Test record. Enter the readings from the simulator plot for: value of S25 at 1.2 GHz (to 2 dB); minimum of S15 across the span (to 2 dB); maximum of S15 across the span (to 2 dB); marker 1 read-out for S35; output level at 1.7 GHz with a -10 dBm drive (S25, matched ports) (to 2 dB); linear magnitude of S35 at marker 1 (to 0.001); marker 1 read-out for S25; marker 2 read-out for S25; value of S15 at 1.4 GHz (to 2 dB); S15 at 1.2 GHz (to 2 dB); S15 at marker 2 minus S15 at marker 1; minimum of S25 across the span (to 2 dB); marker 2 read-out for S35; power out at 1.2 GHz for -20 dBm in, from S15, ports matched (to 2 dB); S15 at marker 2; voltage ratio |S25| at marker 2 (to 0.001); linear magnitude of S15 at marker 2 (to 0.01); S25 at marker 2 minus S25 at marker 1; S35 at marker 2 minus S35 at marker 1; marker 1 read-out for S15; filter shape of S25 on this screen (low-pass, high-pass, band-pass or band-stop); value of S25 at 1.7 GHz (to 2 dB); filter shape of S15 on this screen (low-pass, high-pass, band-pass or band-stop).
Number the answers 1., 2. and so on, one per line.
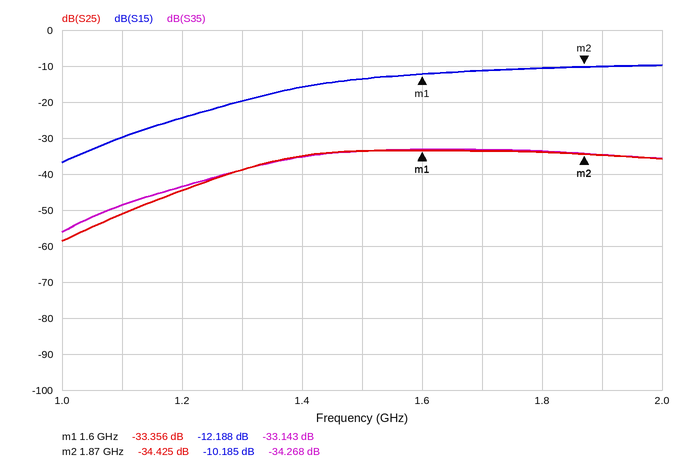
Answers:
1. -44 dB
2. -36 dB
3. -10 dB
4. -33.143 dB
5. -44 dBm
6. 0.022
7. -33.356 dB
8. -34.425 dB
9. -16 dB
10. -24 dB
11. 2.003 dB
12. -58 dB
13. -34.268 dB
14. -44 dBm
15. -10.185 dB
16. 0.019
17. 0.31
18. -1.069 dB
19. -1.125 dB
20. -12.188 dB
21. high-pass
22. -34 dB
23. high-pass
